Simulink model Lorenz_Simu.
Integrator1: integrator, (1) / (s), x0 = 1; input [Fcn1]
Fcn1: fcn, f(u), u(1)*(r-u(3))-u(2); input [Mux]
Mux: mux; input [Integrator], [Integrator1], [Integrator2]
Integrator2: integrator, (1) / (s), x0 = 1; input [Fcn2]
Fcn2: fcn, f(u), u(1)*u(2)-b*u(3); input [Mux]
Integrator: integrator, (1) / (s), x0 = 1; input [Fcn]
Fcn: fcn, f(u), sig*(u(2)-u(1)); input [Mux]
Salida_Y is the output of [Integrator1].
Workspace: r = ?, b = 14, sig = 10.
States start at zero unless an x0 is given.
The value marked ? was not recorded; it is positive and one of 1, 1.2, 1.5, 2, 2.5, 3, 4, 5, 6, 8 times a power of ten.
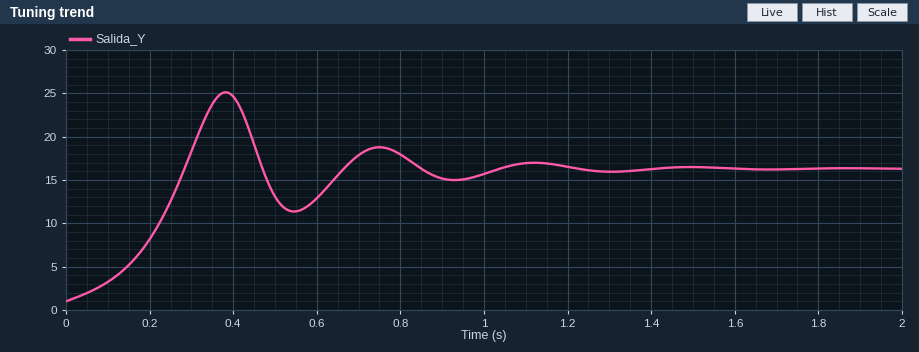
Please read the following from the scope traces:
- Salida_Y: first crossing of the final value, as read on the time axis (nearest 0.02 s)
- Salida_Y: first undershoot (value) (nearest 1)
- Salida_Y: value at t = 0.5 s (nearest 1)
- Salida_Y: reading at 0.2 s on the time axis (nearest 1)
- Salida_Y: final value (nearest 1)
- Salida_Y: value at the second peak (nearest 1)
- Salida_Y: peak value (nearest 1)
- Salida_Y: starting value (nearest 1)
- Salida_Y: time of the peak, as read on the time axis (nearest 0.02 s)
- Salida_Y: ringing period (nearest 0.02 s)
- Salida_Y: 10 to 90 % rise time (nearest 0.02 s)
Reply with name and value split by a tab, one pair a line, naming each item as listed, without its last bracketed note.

Salida_Y: first crossing of the final value, as read on the time axis	0.28 s
Salida_Y: first undershoot (value)	11
Salida_Y: value at t = 0.5 s	13
Salida_Y: reading at 0.2 s on the time axis	8
Salida_Y: final value	16
Salida_Y: value at the second peak	19
Salida_Y: peak value	25
Salida_Y: starting value	1
Salida_Y: time of the peak, as read on the time axis	0.38 s
Salida_Y: ringing period	0.36 s
Salida_Y: 10 to 90 % rise time	0.20 s
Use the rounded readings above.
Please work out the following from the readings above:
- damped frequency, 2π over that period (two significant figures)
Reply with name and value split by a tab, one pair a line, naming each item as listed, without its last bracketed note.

damped frequency, 2π over that period	17 rad/s
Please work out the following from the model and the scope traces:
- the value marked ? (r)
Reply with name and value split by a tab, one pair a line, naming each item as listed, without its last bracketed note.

the value marked ?	20
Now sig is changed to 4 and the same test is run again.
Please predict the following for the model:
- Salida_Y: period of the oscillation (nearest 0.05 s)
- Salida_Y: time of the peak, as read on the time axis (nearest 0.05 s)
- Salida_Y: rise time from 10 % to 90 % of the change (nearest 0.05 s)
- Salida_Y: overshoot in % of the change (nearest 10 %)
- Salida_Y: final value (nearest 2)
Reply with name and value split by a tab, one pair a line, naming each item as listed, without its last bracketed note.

Salida_Y: period of the oscillation	0.45 s
Salida_Y: time of the peak, as read on the time axis	0.50 s
Salida_Y: rise time from 10 % to 90 % of the change	0.25 s
Salida_Y: overshoot in % of the change	70 %
Salida_Y: final value	16
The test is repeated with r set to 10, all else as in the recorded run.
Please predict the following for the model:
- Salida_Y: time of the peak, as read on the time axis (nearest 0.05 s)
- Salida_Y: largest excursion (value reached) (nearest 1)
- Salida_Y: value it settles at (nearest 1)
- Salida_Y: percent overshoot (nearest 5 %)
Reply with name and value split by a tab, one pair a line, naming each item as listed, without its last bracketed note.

Salida_Y: time of the peak, as read on the time axis	0.60 s
Salida_Y: largest excursion (value reached)	14
Salida_Y: value it settles at	11
Salida_Y: percent overshoot	25 %
